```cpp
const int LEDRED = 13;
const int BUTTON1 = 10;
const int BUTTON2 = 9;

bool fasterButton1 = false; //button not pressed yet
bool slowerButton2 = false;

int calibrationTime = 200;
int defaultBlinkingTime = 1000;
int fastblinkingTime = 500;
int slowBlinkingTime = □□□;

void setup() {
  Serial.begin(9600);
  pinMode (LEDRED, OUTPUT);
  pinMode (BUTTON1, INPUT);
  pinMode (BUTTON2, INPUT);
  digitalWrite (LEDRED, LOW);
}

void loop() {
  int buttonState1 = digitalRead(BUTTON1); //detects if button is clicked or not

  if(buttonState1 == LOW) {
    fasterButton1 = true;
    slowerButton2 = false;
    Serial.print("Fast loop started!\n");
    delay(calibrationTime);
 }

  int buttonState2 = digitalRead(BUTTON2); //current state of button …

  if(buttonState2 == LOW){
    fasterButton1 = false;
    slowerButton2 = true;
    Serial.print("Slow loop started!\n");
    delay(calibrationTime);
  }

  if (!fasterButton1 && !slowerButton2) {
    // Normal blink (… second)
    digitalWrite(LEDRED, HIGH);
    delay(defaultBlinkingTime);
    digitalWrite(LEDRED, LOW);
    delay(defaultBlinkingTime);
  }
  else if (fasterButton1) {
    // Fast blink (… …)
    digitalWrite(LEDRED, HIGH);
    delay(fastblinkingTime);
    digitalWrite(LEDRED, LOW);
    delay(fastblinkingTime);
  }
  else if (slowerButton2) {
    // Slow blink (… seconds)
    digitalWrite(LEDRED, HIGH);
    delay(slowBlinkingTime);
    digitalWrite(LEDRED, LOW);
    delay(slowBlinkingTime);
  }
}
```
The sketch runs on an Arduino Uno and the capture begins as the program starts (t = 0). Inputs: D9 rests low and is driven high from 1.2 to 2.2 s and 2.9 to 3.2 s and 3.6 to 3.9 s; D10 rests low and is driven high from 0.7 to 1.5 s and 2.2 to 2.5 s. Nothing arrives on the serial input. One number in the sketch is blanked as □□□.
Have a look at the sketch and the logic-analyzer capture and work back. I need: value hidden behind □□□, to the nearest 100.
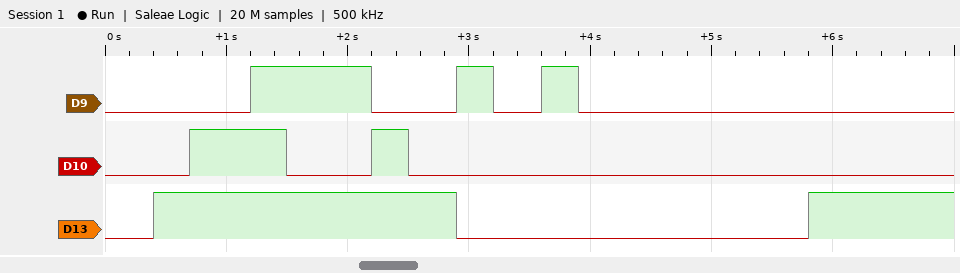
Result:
2500
